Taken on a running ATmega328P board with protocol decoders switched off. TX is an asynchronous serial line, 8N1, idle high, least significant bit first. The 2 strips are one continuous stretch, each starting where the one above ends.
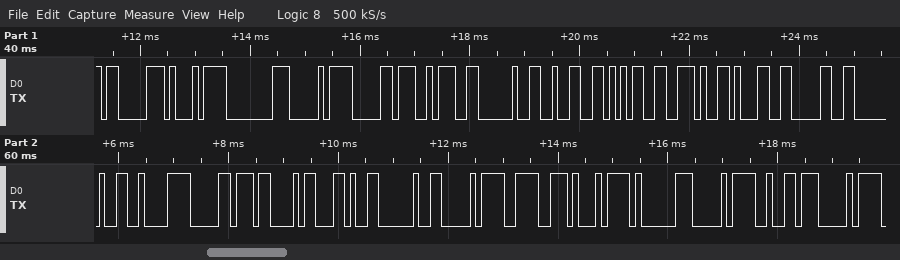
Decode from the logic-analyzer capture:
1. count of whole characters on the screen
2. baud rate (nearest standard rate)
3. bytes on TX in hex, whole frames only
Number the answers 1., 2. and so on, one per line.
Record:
1. 25
2. 9600 baud
3. 83 D1 80 D0 B0 3A 20 32 35 2E 31 30 20 C2 B0 43 2C 20 D0 9E D1 81 D0 B2 D0
